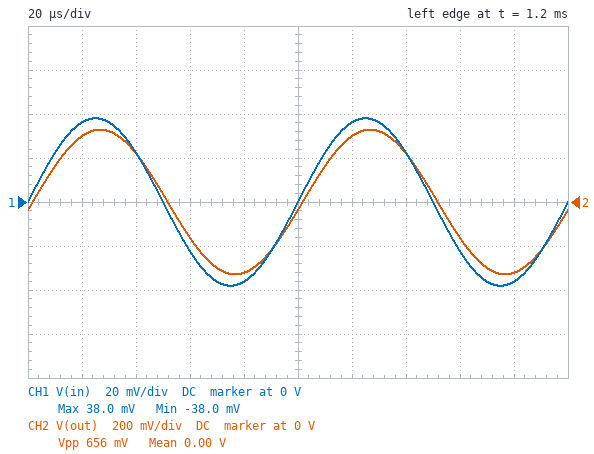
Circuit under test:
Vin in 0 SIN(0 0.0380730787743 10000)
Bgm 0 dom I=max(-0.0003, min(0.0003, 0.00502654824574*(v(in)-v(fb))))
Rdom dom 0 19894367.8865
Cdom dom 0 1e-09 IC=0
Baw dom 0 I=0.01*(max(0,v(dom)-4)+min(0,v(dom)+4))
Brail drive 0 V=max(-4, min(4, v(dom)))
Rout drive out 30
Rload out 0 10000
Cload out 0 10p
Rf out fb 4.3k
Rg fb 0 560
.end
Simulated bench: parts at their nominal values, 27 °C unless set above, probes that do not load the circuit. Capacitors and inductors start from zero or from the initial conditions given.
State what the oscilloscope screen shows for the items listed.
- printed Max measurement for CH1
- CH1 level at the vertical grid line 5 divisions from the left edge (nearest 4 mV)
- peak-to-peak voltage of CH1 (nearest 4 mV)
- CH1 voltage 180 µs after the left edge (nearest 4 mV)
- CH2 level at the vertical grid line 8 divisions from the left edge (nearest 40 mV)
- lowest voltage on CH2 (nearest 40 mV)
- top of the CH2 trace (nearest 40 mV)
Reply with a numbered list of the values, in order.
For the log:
1. 38.0 mV
2. 0 V
3. 76 mV
4. -36 mV
5. -160 mV
6. -320 mV
7. 320 mV
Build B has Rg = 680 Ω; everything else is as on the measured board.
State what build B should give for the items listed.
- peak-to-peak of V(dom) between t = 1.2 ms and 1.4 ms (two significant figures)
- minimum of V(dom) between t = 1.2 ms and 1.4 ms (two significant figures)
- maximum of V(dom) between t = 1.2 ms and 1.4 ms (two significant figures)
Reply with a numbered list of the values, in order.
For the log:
1. 560 mV
2. -280 mV
3. 280 mV
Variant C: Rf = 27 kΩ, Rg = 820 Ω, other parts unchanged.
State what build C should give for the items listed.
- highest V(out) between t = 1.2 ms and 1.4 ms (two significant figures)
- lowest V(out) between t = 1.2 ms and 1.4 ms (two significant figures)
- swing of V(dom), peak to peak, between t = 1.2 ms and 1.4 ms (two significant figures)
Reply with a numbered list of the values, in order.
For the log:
1. 1.2 V
2. -1.2 V
3. 2.4 V
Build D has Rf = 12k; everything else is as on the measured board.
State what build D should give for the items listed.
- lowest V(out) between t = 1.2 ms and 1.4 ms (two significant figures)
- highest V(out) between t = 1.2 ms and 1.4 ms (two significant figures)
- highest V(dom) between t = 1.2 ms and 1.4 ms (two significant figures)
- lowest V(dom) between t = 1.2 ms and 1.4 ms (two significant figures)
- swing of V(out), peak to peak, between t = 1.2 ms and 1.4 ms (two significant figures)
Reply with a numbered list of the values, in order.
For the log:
1. -820 mV
2. 820 mV
3. 830 mV
4. -830 mV
5. 1.6 V
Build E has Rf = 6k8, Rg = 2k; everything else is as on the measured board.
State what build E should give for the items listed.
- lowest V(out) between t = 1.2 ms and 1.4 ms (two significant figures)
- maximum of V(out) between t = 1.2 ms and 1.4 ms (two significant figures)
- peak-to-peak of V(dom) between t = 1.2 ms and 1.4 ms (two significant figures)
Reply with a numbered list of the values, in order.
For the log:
1. -170 mV
2. 170 mV
3. 340 mV
